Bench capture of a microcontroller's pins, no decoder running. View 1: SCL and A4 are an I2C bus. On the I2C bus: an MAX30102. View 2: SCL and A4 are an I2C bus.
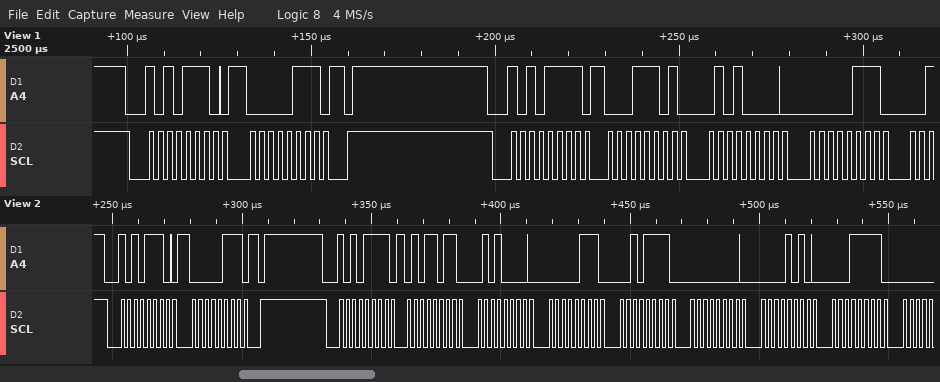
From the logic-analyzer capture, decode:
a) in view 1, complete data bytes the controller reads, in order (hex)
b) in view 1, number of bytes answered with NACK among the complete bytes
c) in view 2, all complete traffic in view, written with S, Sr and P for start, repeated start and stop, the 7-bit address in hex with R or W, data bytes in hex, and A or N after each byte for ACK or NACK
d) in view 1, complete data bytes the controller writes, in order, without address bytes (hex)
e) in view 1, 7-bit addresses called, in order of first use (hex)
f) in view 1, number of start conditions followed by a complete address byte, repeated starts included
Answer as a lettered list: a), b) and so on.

a) 1D 50 07
b) 0
c) S 57W A 07 A P S 57R A 5B A 50 A 07 A 2F A 00 A 0A A 1F A
d) 07
e) 0x57
f) 2
